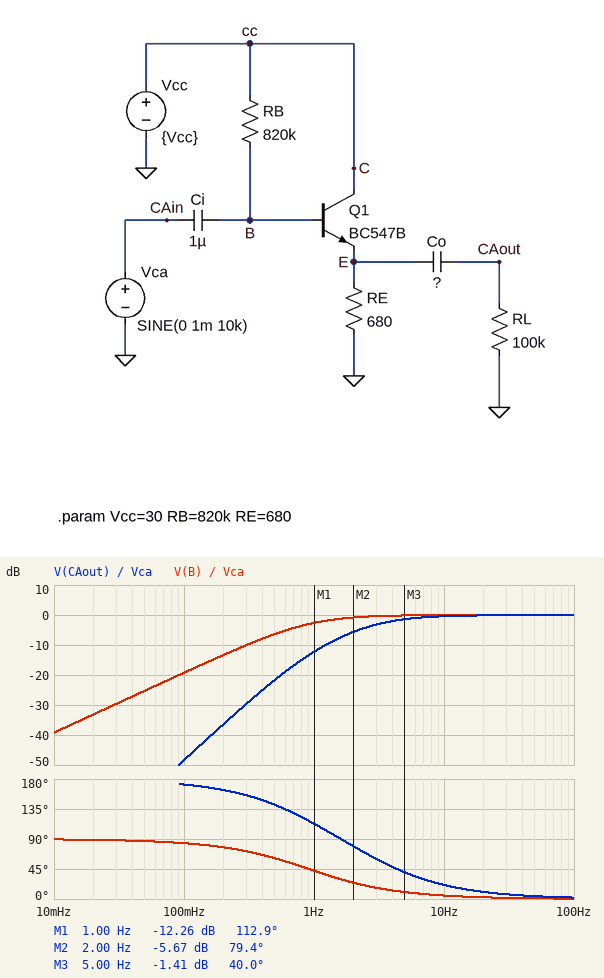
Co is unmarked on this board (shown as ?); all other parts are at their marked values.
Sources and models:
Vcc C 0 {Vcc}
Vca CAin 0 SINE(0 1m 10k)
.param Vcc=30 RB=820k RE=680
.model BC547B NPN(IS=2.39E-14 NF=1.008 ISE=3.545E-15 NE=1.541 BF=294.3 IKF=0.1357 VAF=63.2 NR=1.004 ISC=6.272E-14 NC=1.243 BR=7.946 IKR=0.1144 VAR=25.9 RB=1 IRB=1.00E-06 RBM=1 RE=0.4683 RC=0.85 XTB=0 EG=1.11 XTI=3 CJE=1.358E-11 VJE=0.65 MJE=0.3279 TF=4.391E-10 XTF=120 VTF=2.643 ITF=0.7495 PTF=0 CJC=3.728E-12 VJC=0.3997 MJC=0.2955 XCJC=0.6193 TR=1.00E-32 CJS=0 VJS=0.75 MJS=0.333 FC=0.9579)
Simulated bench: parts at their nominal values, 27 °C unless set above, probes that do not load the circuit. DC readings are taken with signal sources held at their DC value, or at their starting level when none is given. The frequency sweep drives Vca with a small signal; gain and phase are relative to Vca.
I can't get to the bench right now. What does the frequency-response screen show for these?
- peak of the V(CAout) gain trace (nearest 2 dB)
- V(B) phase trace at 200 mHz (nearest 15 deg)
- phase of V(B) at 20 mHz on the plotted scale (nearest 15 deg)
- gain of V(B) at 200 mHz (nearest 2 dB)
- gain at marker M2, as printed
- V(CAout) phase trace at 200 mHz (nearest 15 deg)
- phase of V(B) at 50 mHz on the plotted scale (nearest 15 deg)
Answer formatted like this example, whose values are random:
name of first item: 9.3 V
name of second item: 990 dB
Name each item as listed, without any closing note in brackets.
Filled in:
peak of the V(CAout) gain trace: 0 dB
V(B) phase trace at 200 mHz: 75 deg
phase of V(B) at 20 mHz on the plotted scale: 90 deg
gain of V(B) at 200 mHz: -14 dB
gain at marker M2, as printed: -5.67 dB
V(CAout) phase trace at 200 mHz: 165 deg
phase of V(B) at 50 mHz on the plotted scale: 90 deg
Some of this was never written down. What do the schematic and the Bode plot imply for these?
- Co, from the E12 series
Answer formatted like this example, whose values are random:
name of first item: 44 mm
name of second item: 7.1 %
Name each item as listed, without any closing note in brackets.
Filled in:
Co, from the E12 series: 560 nF
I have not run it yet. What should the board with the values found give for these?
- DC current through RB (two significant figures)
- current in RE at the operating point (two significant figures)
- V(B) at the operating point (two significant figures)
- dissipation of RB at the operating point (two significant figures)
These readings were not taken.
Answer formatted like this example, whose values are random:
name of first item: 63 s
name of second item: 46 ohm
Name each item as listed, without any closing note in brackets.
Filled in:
DC current through RB: 27 µA
current in RE at the operating point: 10 mA
V(B) at the operating point: 7.6 V
dissipation of RB at the operating point: 610 µW
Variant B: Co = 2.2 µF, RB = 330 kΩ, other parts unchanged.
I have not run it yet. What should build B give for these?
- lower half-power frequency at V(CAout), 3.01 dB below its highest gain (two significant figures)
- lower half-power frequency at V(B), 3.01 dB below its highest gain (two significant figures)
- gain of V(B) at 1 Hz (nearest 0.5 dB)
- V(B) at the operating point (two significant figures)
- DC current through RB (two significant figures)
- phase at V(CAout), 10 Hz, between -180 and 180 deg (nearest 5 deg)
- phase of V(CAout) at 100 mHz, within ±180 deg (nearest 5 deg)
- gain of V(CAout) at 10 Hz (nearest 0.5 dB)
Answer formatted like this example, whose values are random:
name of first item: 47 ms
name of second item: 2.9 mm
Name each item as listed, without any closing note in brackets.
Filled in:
lower half-power frequency at V(CAout), 3.01 dB below its highest gain: 1.7 Hz
lower half-power frequency at V(B), 3.01 dB below its highest gain: 1.4 Hz
gain of V(B) at 1 Hz: -4.5 dB
V(B) at the operating point: 13 V
DC current through RB: 53 µA
phase at V(CAout), 10 Hz, between -180 and 180 deg: 10 deg
phase of V(CAout) at 100 mHz, within ±180 deg: 170 deg
gain of V(CAout) at 10 Hz: 0 dB
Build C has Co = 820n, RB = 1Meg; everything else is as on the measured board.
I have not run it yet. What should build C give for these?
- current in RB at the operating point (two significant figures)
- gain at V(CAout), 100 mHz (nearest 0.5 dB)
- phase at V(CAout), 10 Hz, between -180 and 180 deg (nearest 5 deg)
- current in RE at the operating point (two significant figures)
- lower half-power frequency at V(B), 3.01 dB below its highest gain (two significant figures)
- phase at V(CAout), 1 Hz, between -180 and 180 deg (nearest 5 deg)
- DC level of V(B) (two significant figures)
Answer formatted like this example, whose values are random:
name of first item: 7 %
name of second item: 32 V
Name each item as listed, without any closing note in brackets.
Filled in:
current in RB at the operating point: 23 µA
gain at V(CAout), 100 mHz: -44.5 dB
phase at V(CAout), 10 Hz, between -180 and 180 deg: 15 deg
current in RE at the operating point: 8.8 mA
lower half-power frequency at V(B), 3.01 dB below its highest gain: 850 mHz
phase at V(CAout), 1 Hz, between -180 and 180 deg: 105 deg
DC level of V(B): 6.7 V
